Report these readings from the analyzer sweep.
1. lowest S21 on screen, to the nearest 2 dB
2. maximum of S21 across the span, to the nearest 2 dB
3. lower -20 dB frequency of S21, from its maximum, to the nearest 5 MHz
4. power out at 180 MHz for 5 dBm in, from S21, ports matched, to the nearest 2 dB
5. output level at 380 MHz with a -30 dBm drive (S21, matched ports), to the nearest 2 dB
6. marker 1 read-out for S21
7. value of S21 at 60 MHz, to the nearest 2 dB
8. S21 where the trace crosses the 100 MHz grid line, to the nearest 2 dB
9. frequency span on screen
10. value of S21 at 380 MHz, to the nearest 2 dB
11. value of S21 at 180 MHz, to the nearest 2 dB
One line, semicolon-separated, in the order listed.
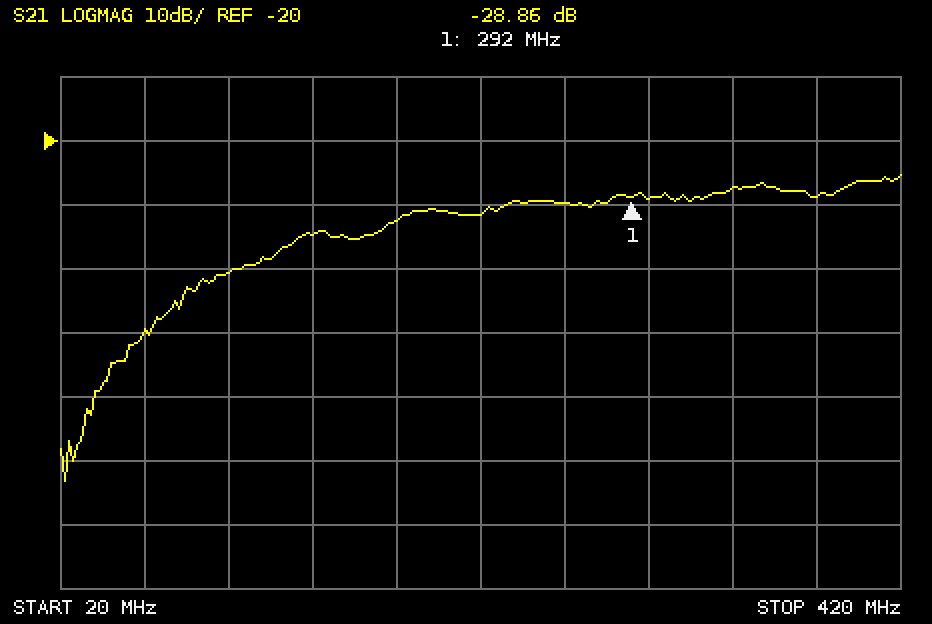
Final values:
-74 dB; -26 dB; 75 MHz; -28 dBm; -58 dBm; -28.86 dB; -50 dB; -40 dB; 400 MHz; -28 dB; -32 dB
